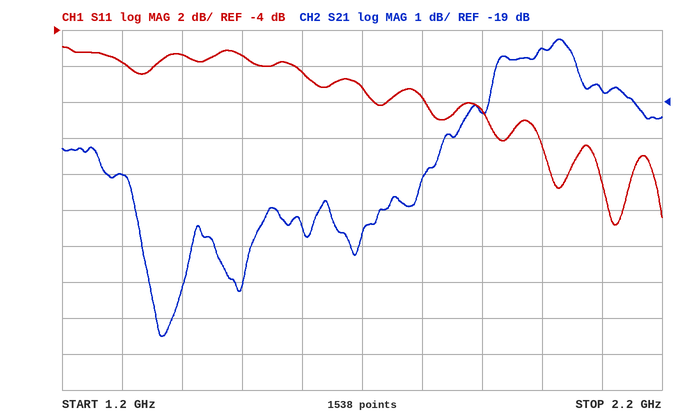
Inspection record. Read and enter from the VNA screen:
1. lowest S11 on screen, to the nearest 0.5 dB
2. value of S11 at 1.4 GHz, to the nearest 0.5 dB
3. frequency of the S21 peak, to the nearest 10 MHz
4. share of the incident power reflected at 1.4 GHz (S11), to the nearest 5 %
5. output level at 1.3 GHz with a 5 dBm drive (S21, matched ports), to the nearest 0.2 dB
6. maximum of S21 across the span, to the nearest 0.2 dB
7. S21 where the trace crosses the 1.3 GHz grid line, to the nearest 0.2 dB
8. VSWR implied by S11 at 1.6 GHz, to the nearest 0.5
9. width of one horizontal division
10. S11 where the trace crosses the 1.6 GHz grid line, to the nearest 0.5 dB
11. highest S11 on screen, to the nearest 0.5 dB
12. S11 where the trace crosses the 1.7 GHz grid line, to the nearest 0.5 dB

-15.0 dB
-5.5 dB
2.03 GHz
30 %
-16.0 dBm
-17.2 dB
-21.0 dB
3.0
100 MHz
-6.5 dB
-5.0 dB
-7.0 dB
